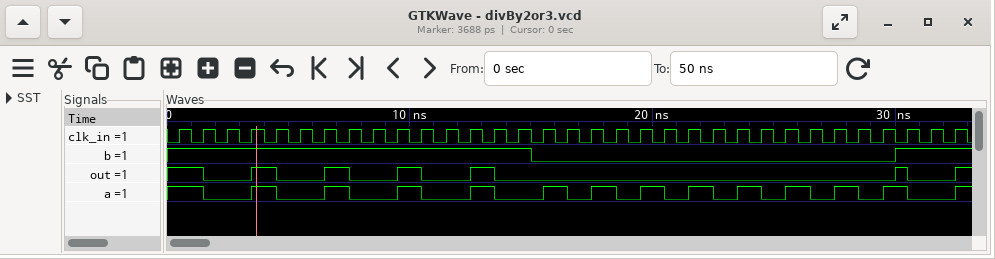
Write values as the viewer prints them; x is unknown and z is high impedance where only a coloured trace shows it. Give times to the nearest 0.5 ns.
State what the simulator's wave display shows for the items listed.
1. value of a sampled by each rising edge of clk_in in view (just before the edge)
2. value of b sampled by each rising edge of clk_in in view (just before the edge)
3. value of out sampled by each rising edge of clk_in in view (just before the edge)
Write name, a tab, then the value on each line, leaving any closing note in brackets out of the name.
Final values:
value of a sampled by each rising edge of clk_in in view	1 1 0 0 1 0 0 1 0 0 1 0 0 1 0 0 1 0 1 0 1 0 1 0 1 0 1 0 1 0 1 0 0
value of b sampled by each rising edge of clk_in in view	1 1 1 1 1 1 1 1 1 1 1 1 1 1 1 0 0 0 0 0 0 0 0 0 0 0 0 0 0 0 1 1 1
value of out sampled by each rising edge of clk_in in view	1 1 0 0 1 0 0 1 0 0 1 0 0 1 0 0 0 0 0 0 0 0 0 0 0 0 0 0 0 0 1 0 0
